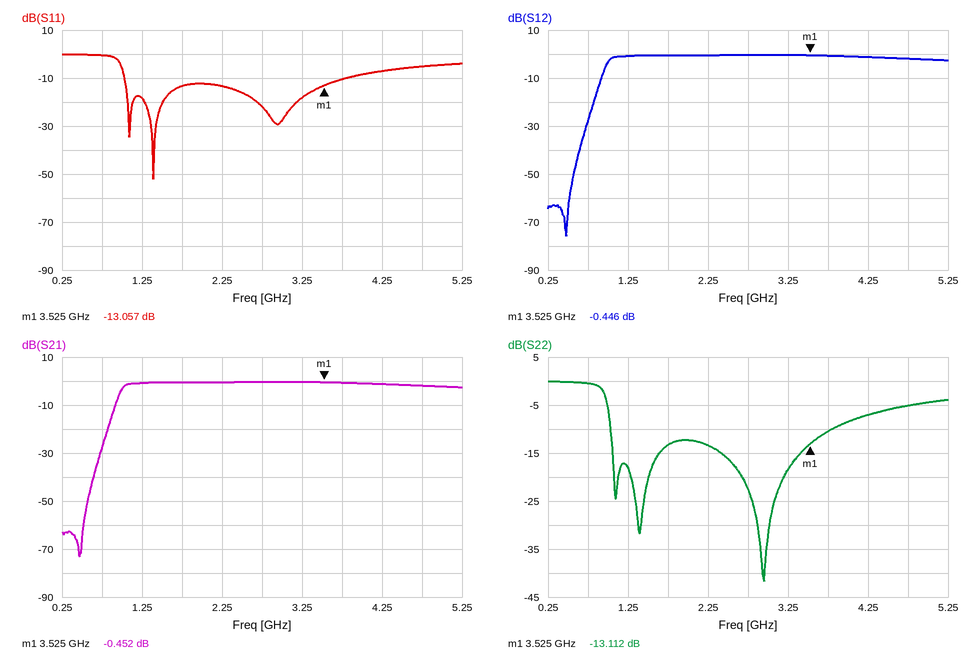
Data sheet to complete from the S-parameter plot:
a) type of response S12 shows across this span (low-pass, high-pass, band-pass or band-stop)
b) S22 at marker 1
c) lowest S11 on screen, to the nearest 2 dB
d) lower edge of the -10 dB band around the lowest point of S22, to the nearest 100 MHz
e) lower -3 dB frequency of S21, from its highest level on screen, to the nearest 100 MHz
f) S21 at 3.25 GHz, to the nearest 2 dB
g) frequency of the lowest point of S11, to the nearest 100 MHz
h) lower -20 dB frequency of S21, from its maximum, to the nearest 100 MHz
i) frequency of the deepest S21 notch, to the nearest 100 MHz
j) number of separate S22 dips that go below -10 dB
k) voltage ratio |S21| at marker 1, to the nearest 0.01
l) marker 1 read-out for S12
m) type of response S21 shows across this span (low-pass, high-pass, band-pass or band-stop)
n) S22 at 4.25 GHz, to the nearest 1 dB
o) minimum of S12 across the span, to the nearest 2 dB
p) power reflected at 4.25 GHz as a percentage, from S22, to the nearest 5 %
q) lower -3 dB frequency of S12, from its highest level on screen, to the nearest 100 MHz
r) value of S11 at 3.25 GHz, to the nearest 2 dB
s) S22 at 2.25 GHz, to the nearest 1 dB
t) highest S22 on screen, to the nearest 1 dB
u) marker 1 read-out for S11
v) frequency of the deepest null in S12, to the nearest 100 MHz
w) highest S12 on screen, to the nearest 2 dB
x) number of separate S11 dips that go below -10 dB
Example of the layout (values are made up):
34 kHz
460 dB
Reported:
high-pass
-13.112 dB
-52 dB
1.0 GHz
1.0 GHz
0 dB
1.4 GHz
800 MHz
500 MHz
3
0.95
-0.446 dB
high-pass
-7 dB
-76 dB
20 %
1.0 GHz
-18 dB
-13 dB
0 dB
-13.057 dB
500 MHz
0 dB
3
